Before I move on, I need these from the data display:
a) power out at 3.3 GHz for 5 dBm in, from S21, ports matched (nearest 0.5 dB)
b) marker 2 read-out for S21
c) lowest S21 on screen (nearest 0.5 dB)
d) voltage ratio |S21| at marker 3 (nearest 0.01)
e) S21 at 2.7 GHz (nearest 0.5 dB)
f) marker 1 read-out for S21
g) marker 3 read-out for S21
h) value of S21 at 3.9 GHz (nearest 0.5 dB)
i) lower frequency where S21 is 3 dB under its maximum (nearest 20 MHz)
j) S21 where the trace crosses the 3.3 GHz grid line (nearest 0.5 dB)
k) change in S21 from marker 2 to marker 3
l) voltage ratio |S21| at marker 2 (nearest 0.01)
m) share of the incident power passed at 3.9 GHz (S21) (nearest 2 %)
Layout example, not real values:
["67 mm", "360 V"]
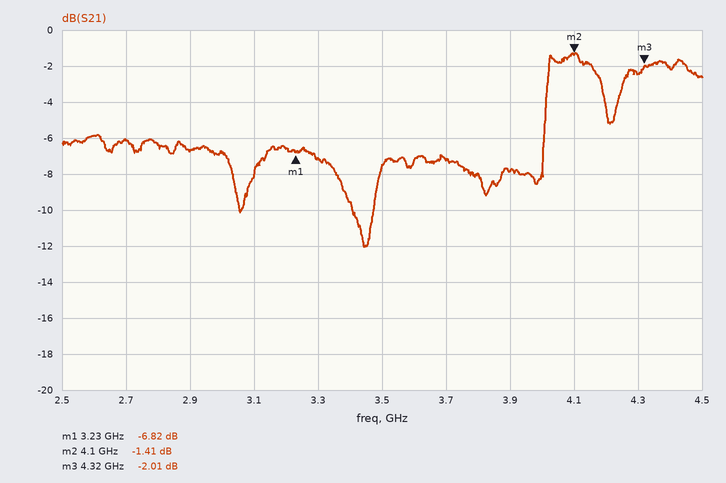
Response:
["-2.0 dBm", "-1.41 dB", "-12.0 dB", "0.79", "-6.0 dB", "-6.82 dB", "-2.01 dB", "-8.0 dB", "4.02 GHz", "-7.0 dB", "-0.60 dB", "0.85", "16 %"]
